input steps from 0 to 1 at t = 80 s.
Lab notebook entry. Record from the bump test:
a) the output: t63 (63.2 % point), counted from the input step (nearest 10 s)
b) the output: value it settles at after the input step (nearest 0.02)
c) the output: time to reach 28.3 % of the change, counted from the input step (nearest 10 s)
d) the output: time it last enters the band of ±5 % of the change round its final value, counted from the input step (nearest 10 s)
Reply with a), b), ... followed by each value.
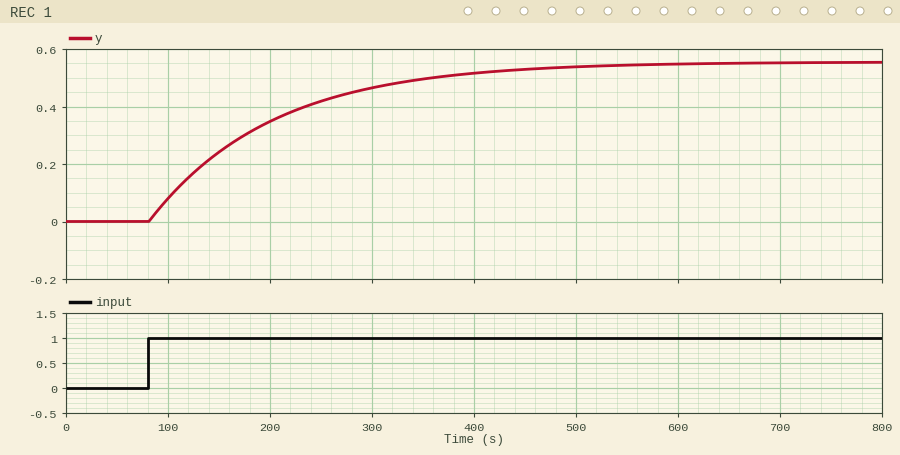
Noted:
a) 120 s
b) 0.56
c) 40 s
d) 360 s
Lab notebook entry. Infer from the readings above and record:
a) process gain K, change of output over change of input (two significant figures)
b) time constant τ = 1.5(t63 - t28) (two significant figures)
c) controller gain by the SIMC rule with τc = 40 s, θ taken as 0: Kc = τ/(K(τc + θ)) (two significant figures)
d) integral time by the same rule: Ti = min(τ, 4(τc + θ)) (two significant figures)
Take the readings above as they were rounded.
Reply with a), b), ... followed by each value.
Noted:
a) 0.56
b) 120 s
c) 5.4
d) 120 s
